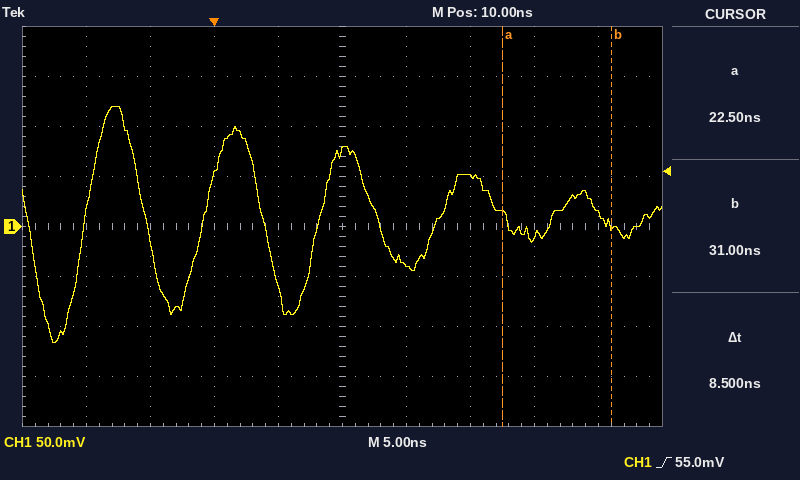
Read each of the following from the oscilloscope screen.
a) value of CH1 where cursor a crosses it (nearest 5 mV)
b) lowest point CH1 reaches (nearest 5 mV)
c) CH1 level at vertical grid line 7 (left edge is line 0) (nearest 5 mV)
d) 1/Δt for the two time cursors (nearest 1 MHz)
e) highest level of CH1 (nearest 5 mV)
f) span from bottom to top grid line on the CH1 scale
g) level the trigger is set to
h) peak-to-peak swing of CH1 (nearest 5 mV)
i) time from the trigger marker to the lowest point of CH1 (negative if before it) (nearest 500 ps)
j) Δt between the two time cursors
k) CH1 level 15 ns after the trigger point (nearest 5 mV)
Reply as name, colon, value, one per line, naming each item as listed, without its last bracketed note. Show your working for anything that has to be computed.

value of CH1 where cursor a crosses it: 15 mV
lowest point CH1 reaches: -115 mV
CH1 level at vertical grid line 7 (left edge is line 0): 50 mV
1/Δt for the two time cursors: 1 / 8.5 ns ≈ 118 MHz
highest level of CH1: 120 mV
span from bottom to top grid line on the CH1 scale: 400 mV
level the trigger is set to: 55.0 mV
peak-to-peak swing of CH1: 120 mV − (-115 mV) = 235 mV
time from the trigger marker to the lowest point of CH1 (negative if before it): -12.5 ns
Δt between the two time cursors: 8.5 ns
CH1 level 15 ns after the trigger point: -40 mV
